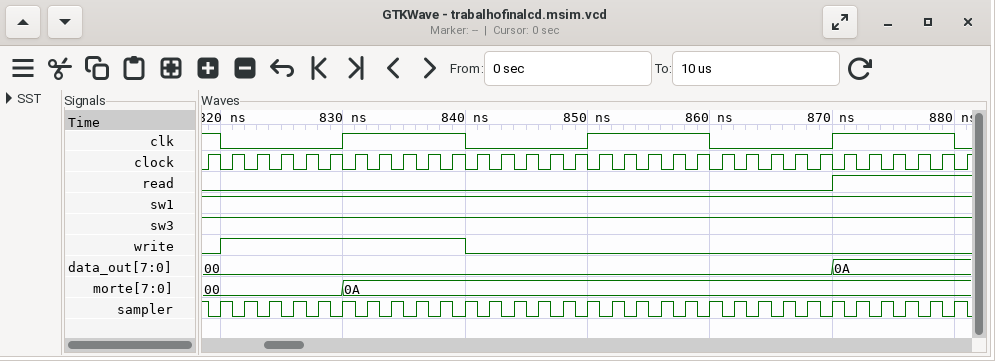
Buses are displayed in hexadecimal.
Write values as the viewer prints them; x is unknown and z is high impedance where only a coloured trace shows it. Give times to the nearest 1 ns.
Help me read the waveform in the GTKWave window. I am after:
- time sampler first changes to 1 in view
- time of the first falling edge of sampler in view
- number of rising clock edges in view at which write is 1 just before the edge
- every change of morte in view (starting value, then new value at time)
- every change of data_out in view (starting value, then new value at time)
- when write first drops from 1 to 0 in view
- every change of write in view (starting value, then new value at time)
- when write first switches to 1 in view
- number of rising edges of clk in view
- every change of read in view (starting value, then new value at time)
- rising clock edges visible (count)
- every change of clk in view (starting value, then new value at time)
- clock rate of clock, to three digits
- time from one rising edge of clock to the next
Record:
820 ns
819 ns
10
00, 0A at 830 ns
00, 0A at 870 ns
840 ns
0, 1 at 820 ns, 0 at 840 ns
820 ns
3
0, 1 at 870 ns
32
1, 0 at 820 ns, 1 at 830 ns, 0 at 840 ns, 1 at 850 ns, 0 at 860 ns, 1 at 870 ns, 0 at 880 ns
500 MHz
2 ns
